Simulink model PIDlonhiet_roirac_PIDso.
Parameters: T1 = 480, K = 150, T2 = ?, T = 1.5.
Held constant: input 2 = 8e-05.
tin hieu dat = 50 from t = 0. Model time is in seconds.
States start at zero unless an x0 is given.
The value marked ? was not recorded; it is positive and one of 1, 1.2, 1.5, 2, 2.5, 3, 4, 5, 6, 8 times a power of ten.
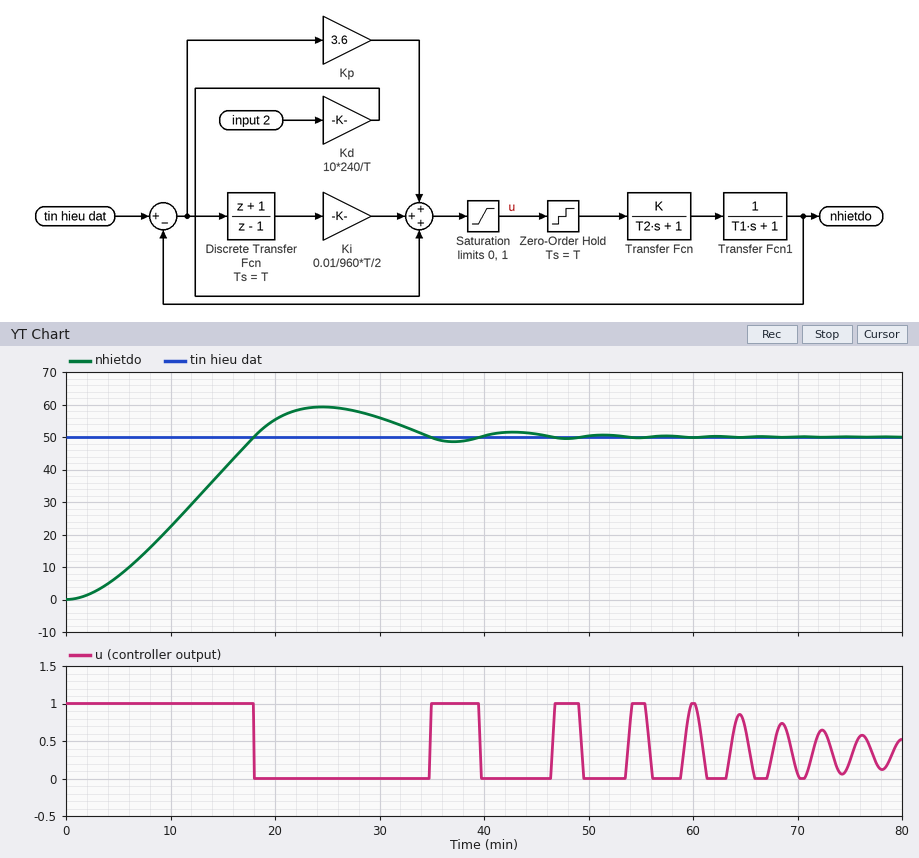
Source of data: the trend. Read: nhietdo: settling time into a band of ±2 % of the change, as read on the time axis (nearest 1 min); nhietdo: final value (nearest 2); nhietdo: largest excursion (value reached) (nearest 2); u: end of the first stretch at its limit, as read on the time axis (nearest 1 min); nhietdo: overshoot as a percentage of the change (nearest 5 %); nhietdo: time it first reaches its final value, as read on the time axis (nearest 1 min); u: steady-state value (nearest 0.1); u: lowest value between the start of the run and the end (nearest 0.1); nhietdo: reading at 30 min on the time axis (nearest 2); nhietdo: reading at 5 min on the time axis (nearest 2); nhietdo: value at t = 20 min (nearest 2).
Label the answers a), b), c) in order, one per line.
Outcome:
a) 45 min
b) 50
c) 60
d) 18 min
e) 20 %
f) 18 min
g) 0.3
h) 0.0
i) 56
j) 8
k) 56
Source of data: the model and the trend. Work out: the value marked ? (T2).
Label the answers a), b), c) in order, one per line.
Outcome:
a) 1500
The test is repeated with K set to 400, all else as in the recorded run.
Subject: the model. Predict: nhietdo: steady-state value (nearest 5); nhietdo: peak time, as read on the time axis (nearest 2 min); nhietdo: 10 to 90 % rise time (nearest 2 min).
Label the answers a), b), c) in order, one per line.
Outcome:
a) 50
b) 18 min
c) 6 min
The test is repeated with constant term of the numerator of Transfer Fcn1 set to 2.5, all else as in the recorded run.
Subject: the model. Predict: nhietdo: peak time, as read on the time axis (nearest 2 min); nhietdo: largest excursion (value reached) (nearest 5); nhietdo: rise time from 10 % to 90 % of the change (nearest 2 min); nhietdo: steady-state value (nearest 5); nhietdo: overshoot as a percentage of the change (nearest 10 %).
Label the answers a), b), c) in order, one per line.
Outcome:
a) 18 min
b) 80
c) 6 min
d) 50
e) 60 %
